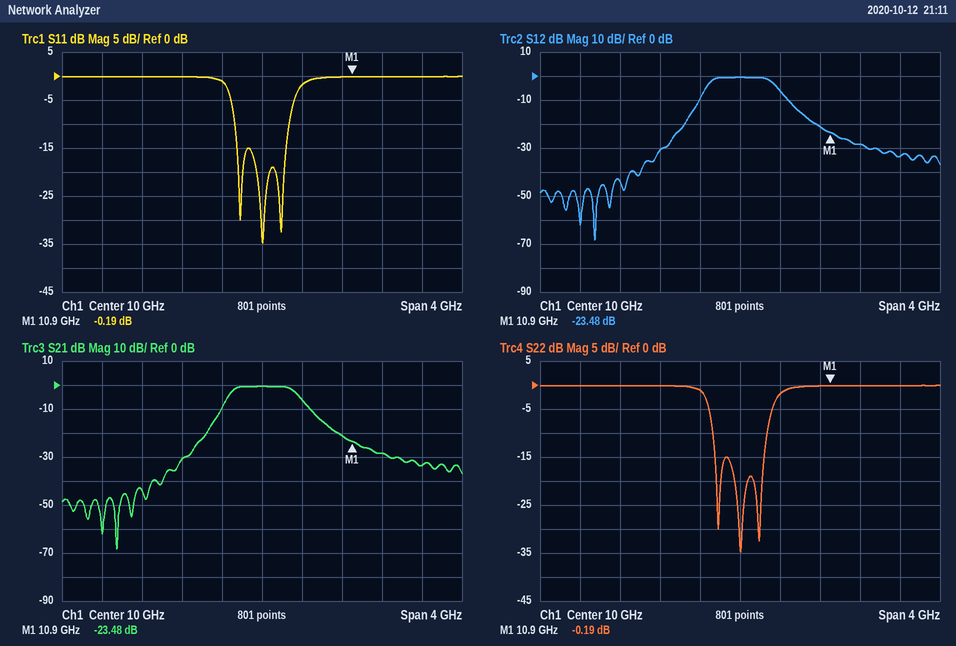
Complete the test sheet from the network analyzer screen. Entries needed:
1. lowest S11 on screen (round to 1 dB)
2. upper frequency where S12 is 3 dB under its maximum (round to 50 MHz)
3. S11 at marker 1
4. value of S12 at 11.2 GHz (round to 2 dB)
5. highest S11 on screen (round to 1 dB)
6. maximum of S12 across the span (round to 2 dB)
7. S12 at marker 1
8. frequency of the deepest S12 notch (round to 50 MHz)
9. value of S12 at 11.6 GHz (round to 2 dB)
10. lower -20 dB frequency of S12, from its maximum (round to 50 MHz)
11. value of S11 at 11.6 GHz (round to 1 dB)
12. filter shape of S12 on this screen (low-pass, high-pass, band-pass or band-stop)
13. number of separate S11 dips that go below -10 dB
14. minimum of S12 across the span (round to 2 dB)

-35 dB
10.35 GHz
-0.19 dB
-28 dB
0 dB
0 dB
-23.48 dB
8.55 GHz
-34 dB
9.45 GHz
0 dB
band-pass
3
-68 dB
